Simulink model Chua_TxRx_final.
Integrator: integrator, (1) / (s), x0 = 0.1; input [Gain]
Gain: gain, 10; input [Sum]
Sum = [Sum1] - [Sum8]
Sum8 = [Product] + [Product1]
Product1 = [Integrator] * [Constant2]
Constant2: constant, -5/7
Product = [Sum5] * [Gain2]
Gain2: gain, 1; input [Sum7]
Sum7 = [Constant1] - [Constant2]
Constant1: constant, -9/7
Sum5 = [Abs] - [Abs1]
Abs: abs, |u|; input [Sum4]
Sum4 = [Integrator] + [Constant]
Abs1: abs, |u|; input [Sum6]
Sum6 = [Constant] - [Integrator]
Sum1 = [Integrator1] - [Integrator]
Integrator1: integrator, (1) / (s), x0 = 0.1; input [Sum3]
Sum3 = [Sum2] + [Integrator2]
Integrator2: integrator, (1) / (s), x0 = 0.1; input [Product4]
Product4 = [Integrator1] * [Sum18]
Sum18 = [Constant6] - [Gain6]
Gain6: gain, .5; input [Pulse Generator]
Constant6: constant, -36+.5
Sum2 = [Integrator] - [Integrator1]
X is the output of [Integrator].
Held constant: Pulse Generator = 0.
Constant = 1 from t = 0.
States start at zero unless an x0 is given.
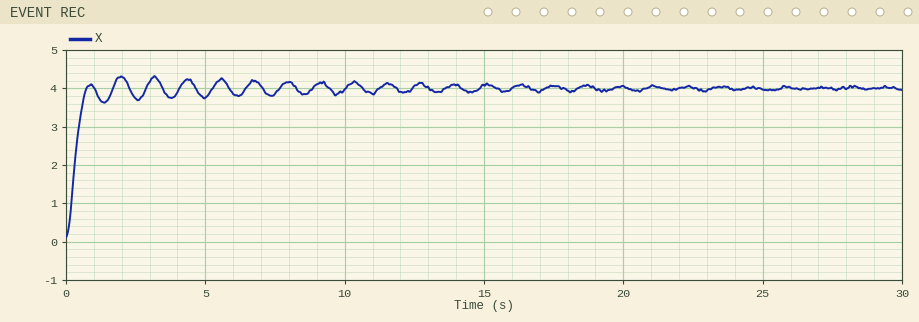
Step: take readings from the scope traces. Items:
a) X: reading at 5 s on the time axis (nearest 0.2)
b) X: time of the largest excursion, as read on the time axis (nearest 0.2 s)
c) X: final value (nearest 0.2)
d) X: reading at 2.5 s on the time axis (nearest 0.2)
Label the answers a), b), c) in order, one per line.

a) 3.8
b) 2.0 s
c) 4.0
d) 3.8
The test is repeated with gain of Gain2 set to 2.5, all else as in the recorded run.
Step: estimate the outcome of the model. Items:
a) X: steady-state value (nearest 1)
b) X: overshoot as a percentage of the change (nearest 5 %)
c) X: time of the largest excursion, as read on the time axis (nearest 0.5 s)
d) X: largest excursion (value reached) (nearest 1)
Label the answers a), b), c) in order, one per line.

a) 10
b) 10 %
c) 2.0 s
d) 11
